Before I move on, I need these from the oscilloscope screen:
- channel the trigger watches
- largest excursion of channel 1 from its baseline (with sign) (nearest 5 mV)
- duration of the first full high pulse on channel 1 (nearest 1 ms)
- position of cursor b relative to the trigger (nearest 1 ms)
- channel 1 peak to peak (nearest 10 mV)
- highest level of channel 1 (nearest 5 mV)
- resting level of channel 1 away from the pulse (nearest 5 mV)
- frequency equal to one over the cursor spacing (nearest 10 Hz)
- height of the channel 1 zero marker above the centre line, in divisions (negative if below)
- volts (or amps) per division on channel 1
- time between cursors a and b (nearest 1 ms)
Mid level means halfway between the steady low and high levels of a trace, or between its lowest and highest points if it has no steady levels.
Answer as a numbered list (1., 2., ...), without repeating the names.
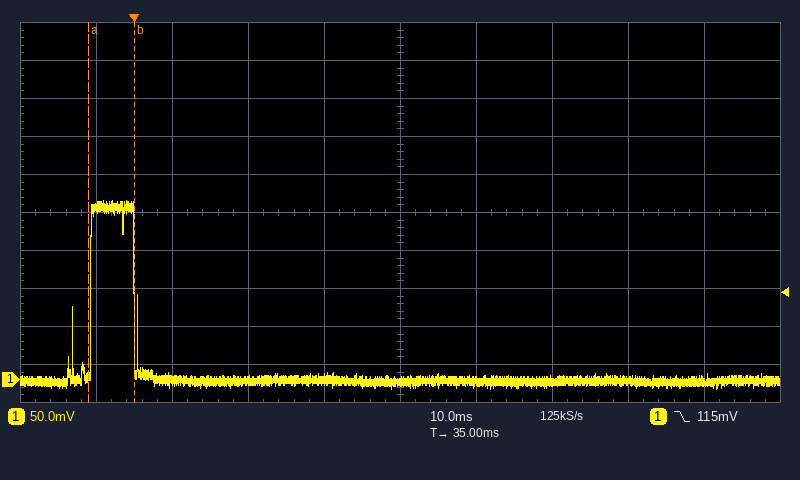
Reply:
1. channel 1
2. +235 mV
3. 6 ms
4. 0 ms
5. 250 mV
6. 235 mV
7. 0 mV
8. 170 Hz
9. -4.4 div
10. 50 mV
11. 6 ms
